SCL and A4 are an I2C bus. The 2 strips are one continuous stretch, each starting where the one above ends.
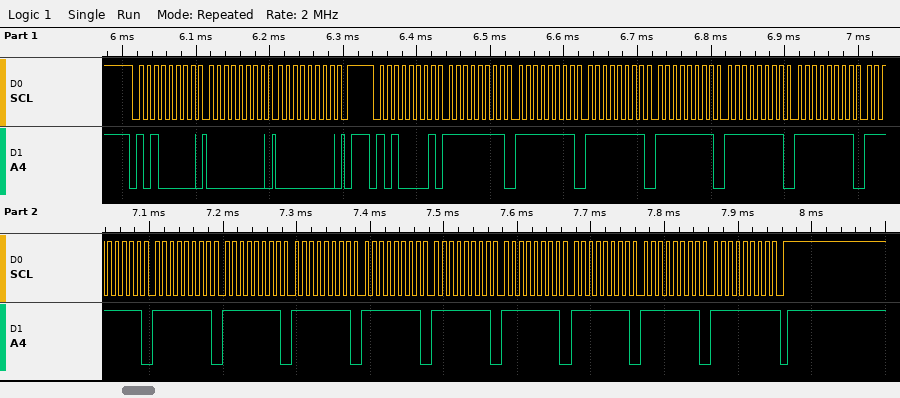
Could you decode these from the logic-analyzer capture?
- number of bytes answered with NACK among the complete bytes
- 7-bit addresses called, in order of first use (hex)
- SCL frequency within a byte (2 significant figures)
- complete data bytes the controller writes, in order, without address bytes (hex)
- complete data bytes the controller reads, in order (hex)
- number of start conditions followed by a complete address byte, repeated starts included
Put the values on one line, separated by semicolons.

1; 0x50; 100 kHz; 00 00; FF FF FF FF FF FF FF FF FF FF FF FF FF FF FF FF; 2
